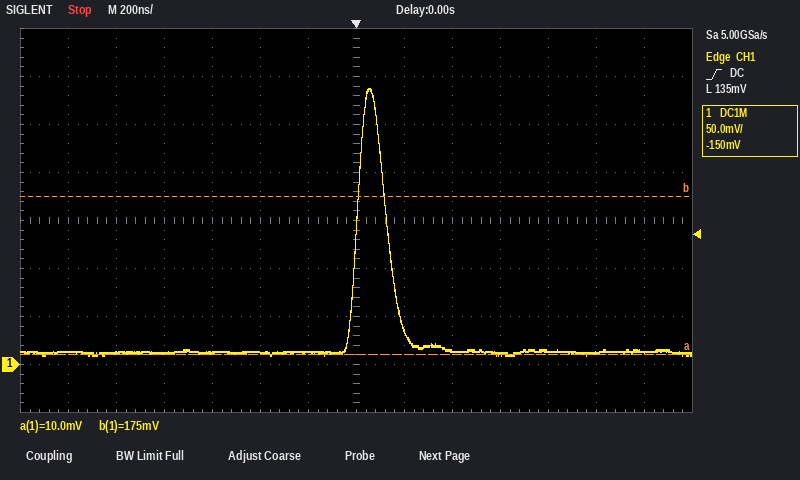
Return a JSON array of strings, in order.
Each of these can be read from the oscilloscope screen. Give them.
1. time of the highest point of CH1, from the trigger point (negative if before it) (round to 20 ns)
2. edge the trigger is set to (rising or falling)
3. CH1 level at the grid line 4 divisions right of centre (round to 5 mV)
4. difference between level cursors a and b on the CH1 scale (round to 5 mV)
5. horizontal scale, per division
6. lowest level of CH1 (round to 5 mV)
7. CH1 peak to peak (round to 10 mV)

["+60 ns", "rising", "15 mV", "165 mV", "200 ns", "10 mV", "280 mV"]
